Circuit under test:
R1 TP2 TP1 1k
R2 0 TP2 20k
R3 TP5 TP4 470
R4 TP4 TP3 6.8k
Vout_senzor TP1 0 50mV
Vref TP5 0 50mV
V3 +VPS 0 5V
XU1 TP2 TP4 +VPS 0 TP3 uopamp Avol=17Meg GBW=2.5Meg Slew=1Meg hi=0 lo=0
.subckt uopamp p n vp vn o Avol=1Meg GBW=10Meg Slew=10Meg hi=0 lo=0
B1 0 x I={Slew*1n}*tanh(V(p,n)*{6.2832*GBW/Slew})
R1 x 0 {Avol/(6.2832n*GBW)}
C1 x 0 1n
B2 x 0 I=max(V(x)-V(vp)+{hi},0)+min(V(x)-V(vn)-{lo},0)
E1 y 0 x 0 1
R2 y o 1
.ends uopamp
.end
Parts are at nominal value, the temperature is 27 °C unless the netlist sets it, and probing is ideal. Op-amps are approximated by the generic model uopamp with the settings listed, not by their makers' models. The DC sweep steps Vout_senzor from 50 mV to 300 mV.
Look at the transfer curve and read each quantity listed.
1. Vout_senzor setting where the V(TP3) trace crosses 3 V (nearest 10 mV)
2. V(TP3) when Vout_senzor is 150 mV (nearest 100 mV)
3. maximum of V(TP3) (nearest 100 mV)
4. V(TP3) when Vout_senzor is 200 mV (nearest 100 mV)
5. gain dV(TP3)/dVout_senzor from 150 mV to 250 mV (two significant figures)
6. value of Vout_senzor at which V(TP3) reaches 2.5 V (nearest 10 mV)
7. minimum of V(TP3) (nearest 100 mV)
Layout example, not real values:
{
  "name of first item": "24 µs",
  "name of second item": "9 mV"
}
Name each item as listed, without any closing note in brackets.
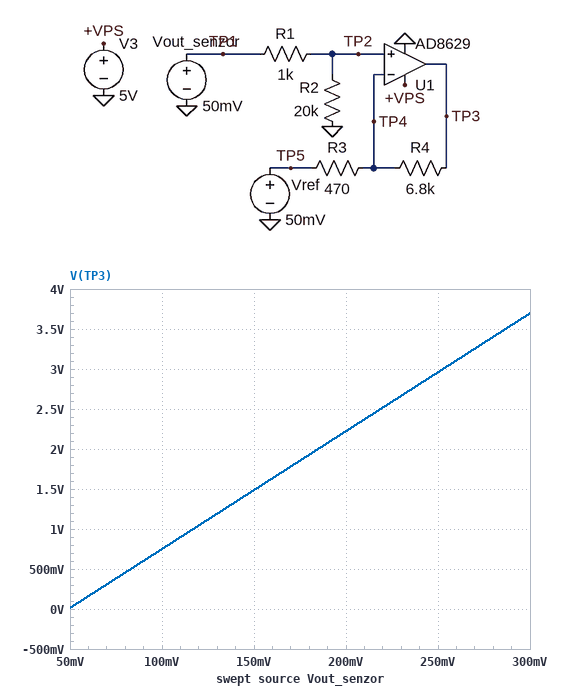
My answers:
{
  "Vout_senzor setting where the V(TP3) trace crosses 3 V": "250 mV",
  "V(TP3) when Vout_senzor is 150 mV": "1.5 V",
  "maximum of V(TP3)": "3.7 V",
  "V(TP3) when Vout_senzor is 200 mV": "2.2 V",
  "gain dV(TP3)/dVout_senzor from 150 mV to 250 mV": "15 V/V",
  "value of Vout_senzor at which V(TP3) reaches 2.5 V": "220 mV",
  "minimum of V(TP3)": "0 V"
}
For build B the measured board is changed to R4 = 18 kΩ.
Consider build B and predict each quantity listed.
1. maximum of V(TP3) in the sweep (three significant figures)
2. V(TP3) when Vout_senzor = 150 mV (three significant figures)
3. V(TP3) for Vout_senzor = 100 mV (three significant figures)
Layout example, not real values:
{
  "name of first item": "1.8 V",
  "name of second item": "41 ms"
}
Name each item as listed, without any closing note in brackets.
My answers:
{
  "maximum of V(TP3) in the sweep": "5.00 V",
  "V(TP3) when Vout_senzor = 150 mV": "3.70 V",
  "V(TP3) for Vout_senzor = 100 mV": "1.83 V"
}
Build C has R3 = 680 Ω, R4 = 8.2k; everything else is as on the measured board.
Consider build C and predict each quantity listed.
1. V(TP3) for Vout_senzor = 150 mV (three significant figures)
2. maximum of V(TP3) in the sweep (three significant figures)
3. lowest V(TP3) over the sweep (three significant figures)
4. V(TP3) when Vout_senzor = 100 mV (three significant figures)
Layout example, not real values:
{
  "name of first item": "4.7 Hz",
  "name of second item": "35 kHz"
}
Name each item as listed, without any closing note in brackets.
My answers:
{
  "V(TP3) for Vout_senzor = 150 mV": "1.26 V",
  "maximum of V(TP3) in the sweep": "3.13 V",
  "lowest V(TP3) over the sweep": "18.9 mV",
  "V(TP3) when Vout_senzor = 100 mV": "641 mV"
}
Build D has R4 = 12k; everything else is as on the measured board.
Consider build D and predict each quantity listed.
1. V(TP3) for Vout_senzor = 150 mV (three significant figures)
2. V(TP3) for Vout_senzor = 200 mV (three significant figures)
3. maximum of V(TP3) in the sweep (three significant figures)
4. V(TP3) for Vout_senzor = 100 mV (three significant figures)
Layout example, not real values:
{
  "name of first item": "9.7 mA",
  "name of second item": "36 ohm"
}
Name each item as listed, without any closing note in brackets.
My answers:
{
  "V(TP3) for Vout_senzor = 150 mV": "2.51 V",
  "V(TP3) for Vout_senzor = 200 mV": "3.78 V",
  "maximum of V(TP3) in the sweep": "5.00 V",
  "V(TP3) for Vout_senzor = 100 mV": "1.25 V"
}
